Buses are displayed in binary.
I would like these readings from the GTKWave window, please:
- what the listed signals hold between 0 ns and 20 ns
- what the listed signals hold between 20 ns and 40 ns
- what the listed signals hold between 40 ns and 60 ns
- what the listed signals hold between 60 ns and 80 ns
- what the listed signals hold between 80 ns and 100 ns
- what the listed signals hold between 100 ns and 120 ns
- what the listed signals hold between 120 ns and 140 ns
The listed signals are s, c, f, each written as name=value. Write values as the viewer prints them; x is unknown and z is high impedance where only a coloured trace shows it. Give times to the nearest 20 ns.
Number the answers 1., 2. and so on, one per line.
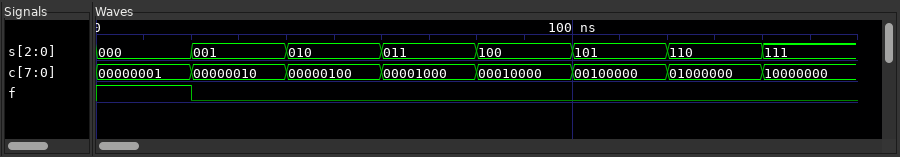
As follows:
1. s=000, c=00000001, f=1
2. s=001, c=00000010, f=0
3. s=010, c=00000100, f=0
4. s=011, c=00001000, f=0
5. s=100, c=00010000, f=0
6. s=101, c=00100000, f=0
7. s=110, c=01000000, f=0
